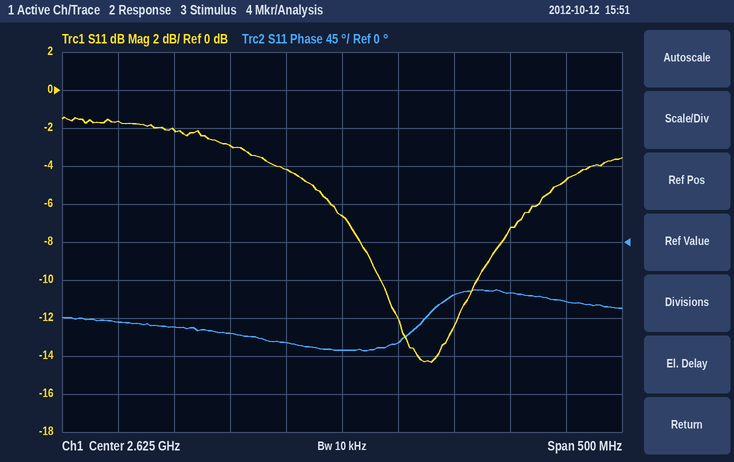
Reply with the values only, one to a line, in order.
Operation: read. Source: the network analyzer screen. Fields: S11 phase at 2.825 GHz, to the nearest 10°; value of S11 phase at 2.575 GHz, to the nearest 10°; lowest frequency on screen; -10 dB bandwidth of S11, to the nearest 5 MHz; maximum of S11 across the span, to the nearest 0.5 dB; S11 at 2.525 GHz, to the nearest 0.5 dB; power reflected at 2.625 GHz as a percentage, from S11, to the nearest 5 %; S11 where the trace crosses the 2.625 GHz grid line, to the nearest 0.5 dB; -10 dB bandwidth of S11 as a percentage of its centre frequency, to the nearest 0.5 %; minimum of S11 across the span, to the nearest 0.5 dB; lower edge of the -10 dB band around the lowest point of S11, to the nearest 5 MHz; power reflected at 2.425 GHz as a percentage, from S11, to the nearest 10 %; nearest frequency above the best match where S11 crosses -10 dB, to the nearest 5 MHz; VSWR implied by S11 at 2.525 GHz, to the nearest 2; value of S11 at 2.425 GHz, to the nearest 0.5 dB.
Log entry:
-70°
-120°
2.375 GHz
85 MHz
-1.5 dB
-3.0 dB
20 %
-6.5 dB
3.0 %
-14.5 dB
2.660 GHz
70 %
2.745 GHz
6
-1.5 dB
